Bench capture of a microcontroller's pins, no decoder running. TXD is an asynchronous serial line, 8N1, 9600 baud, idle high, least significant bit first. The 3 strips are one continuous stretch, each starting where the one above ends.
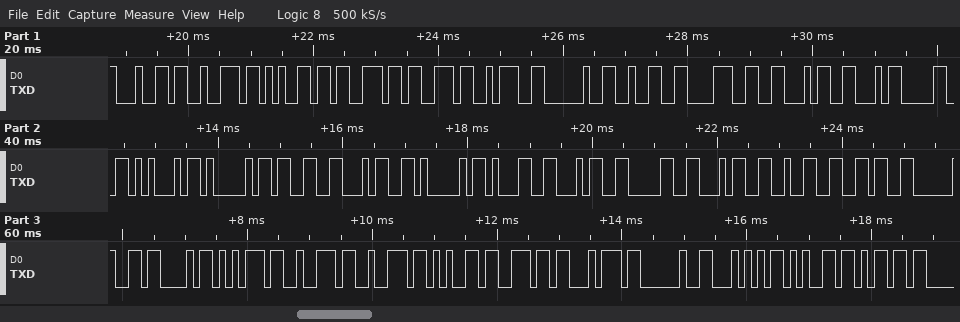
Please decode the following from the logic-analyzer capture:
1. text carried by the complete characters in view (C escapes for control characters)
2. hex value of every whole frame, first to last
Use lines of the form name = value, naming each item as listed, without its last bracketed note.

text carried by the complete characters in view = "dress: 28FF0EA34A140426 Current Tem"
hex value of every whole frame, first to last = 64 72 65 73 73 3A 20 32 38 46 46 30 45 41 33 34 41 31 34 30 34 32 36 20 43 75 72 72 65 6E 74 20 54 65 6D
